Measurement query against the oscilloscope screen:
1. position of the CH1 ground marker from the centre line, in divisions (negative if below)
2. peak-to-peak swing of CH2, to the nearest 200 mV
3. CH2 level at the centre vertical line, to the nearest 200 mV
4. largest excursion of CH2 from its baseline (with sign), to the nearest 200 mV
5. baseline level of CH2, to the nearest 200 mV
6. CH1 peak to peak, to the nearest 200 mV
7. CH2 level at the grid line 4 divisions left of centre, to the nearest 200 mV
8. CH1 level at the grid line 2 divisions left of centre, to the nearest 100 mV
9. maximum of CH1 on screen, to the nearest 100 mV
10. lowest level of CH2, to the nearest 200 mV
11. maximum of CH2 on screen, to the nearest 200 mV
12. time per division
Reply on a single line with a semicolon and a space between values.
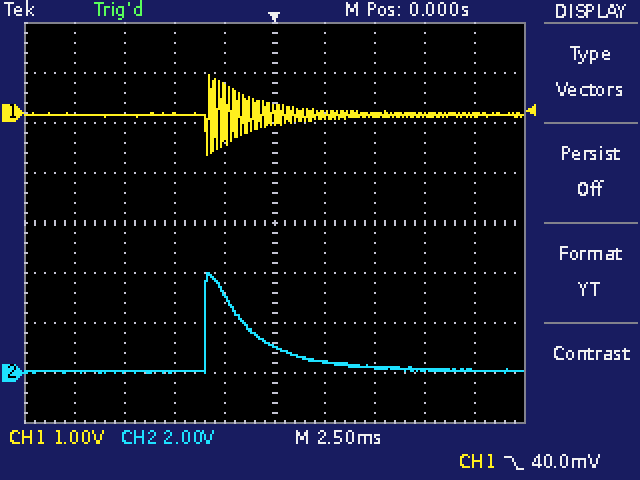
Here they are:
+2.2 div; 4.0 V; 1.0 V; +4.0 V; 0.0 V; 1.6 V; 0.0 V; 0.0 V; 800 mV; 0.0 V; 4.0 V; 2.5 ms
